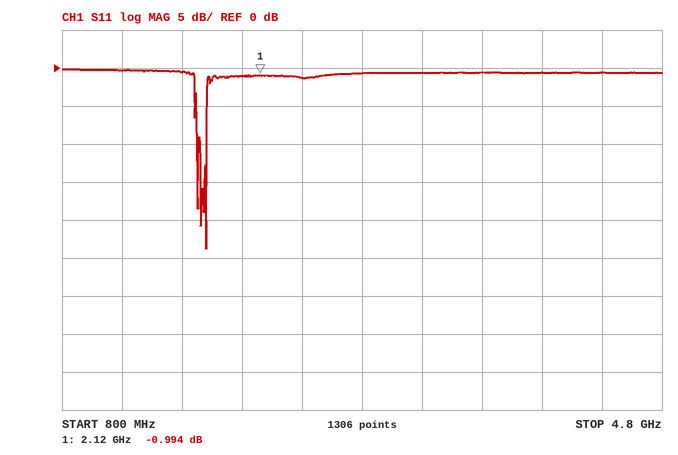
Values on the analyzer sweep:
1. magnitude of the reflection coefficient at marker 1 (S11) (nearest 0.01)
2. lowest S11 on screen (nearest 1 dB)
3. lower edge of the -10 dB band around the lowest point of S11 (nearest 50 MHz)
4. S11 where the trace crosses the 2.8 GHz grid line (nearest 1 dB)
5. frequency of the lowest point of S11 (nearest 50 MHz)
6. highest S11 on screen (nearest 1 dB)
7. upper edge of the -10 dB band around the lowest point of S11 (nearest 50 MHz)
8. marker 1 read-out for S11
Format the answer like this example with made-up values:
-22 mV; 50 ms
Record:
0.89; -24 dB; 1.70 GHz; -1 dB; 1.75 GHz; 0 dB; 1.75 GHz; -0.994 dB
